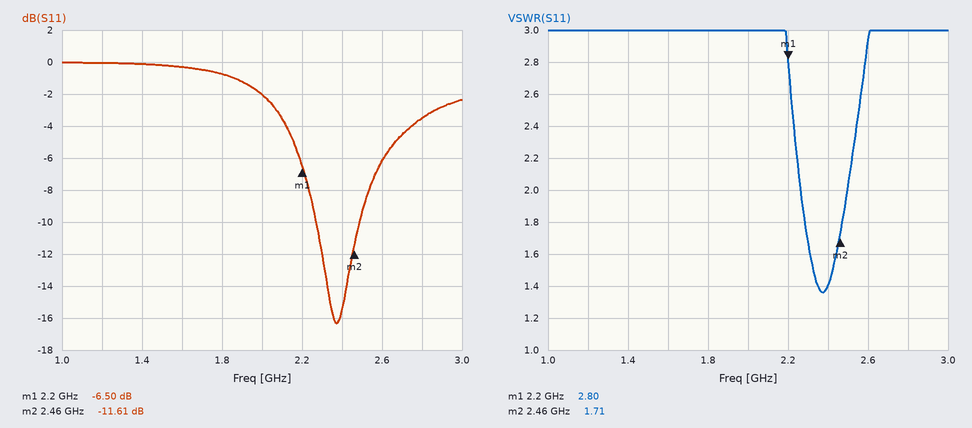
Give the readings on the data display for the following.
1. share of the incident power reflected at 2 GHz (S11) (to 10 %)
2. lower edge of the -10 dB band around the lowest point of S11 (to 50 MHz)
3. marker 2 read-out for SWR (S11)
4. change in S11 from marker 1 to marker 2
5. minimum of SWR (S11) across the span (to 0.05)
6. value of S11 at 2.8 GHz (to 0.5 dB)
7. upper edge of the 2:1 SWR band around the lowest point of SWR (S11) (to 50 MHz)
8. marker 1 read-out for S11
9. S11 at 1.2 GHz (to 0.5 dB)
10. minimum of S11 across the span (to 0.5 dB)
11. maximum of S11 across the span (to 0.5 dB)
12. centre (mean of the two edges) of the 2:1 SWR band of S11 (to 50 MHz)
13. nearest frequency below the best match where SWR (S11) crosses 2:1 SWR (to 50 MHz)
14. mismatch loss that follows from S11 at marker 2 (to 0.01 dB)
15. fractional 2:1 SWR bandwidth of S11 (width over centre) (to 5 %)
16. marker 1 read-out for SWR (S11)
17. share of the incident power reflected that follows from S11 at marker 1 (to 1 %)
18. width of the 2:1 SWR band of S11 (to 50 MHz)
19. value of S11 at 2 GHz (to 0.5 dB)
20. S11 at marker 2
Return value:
60 %
2.25 GHz
1.71
-5.11 dB
1.35
-3.5 dB
2.50 GHz
-6.50 dB
0.0 dB
-16.5 dB
0.0 dB
2.40 GHz
2.25 GHz
0.31 dB
10 %
2.80
22 %
250 MHz
-2.0 dB
-11.61 dB
